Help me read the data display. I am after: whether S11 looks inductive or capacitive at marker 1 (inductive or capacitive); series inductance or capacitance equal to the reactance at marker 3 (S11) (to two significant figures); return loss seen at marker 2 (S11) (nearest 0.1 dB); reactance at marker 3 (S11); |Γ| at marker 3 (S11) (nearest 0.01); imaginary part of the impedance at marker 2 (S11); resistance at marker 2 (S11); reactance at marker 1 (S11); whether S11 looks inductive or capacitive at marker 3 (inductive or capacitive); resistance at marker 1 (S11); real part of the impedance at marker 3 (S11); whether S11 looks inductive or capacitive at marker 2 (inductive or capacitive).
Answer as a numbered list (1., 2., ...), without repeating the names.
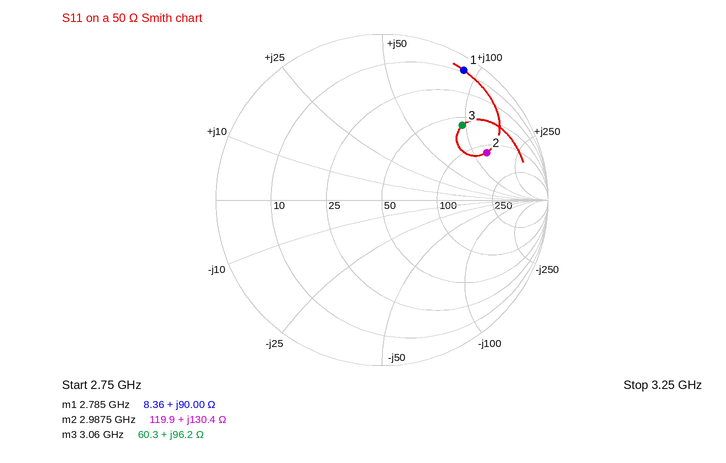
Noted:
1. inductive
2. 5.0 nH
3. 3.2 dB
4. +96.2 Ω
5. 0.66
6. +130.4 Ω
7. 119.9 Ω
8. +90.00 Ω
9. inductive
10. 8.36 Ω
11. 60.3 Ω
12. inductive
